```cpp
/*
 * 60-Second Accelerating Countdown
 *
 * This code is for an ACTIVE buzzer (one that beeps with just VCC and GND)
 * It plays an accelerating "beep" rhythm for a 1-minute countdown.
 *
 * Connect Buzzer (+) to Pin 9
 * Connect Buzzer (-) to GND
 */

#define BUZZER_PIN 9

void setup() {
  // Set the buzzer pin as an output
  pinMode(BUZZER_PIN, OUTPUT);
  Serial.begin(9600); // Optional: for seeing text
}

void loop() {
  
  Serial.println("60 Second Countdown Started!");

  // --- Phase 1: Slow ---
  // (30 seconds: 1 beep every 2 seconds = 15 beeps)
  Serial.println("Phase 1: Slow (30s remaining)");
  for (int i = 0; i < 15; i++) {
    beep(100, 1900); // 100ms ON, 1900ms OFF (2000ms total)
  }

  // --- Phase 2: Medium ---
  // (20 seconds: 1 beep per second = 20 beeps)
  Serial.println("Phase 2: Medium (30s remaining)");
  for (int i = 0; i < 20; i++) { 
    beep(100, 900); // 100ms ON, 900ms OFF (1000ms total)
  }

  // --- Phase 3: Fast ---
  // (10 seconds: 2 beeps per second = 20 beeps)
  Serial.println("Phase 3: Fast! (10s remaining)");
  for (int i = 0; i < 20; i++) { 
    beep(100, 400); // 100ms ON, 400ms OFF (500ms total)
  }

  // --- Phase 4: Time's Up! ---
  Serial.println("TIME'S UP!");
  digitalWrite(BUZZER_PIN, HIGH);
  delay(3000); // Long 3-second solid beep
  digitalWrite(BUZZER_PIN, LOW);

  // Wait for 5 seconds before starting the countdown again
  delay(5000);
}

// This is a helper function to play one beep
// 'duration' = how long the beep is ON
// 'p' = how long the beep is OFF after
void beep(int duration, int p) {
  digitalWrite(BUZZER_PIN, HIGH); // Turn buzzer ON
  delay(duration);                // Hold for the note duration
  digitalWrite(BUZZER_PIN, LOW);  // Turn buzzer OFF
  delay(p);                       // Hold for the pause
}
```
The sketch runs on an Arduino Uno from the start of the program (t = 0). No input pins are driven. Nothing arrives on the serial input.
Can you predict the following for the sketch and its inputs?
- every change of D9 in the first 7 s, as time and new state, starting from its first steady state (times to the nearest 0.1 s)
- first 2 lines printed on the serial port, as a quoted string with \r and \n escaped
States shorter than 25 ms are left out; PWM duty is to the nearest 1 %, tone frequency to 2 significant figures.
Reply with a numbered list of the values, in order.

1. 0 s high; 0.1 s low; 2 s high; 2.1 s low; 4 s high; 4.1 s low; 6 s high; 6.1 s low
2. "60 Second Countdown Started!\r\nPhase 1: Slow (30s remaining)\r\n"
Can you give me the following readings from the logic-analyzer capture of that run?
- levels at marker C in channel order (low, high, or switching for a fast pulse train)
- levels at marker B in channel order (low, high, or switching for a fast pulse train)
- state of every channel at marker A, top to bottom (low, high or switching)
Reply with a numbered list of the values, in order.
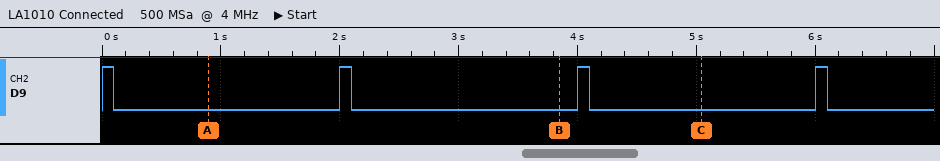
1. D9 low
2. D9 low
3. D9 low
